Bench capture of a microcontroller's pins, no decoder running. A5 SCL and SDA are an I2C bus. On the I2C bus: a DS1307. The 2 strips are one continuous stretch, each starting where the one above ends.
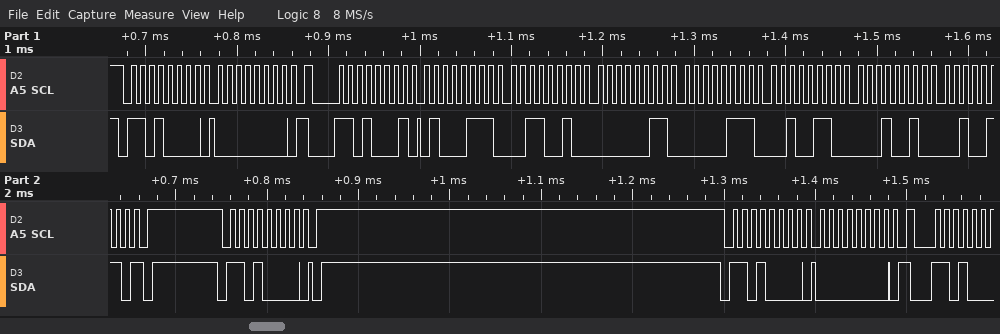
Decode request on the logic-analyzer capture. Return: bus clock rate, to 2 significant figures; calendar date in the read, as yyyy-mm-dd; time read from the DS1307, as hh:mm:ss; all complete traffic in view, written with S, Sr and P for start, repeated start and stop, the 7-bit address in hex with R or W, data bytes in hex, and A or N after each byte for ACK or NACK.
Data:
100 kHz
2026-12-26
03:32:47
S 68W A 00 A Sr 68R A 47 A 32 A 03 A 07 A 26 A 12 A 26 N P S 68W A P S 68W A 00 A
